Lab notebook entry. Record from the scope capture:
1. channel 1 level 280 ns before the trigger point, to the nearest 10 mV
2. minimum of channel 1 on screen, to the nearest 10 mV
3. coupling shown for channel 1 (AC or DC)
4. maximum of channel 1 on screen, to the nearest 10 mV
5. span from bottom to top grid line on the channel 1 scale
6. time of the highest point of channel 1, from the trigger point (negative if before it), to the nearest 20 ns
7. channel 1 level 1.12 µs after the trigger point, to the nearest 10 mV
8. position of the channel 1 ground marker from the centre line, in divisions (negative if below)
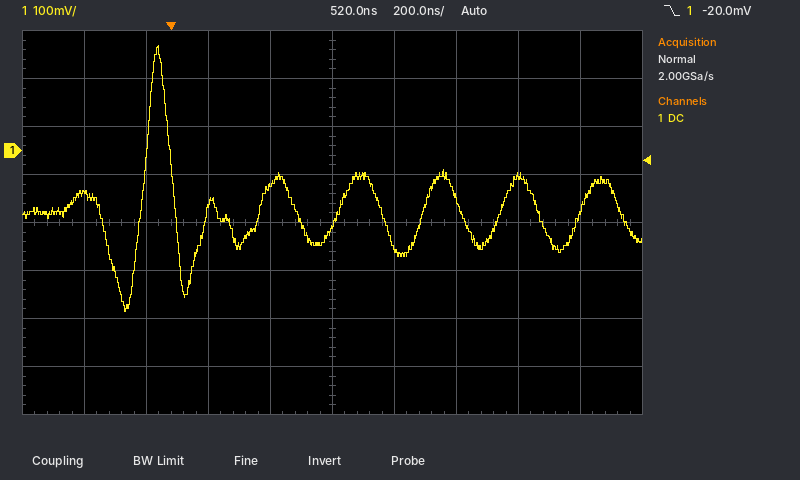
-90 mV
-340 mV
DC
220 mV
800 mV
-40 ns
-50 mV
+1.5 div
